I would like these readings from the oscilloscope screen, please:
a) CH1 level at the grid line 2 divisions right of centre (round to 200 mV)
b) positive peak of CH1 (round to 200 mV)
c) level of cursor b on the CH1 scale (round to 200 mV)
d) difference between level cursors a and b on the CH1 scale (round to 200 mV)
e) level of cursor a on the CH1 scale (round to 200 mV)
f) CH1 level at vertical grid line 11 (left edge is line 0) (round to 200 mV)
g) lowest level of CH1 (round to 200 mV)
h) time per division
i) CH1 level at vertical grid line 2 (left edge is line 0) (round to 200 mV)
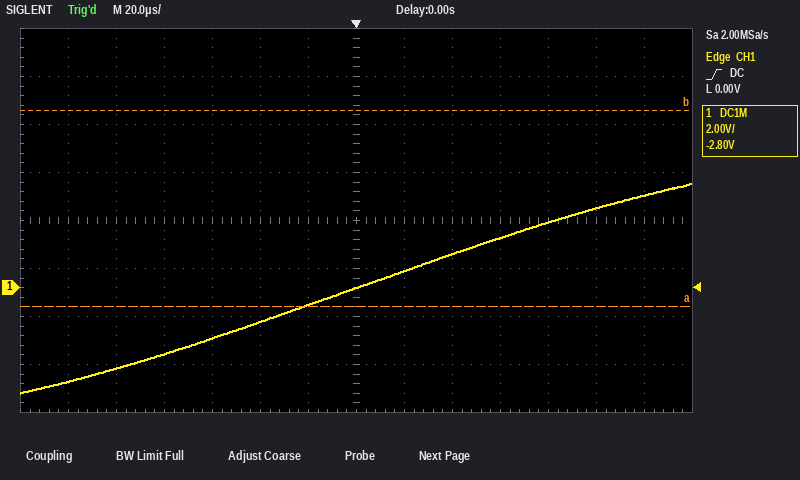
1.4 V
4.4 V
7.4 V
8.2 V
-800 mV
2.8 V
-4.4 V
20 µs
-3.4 V
